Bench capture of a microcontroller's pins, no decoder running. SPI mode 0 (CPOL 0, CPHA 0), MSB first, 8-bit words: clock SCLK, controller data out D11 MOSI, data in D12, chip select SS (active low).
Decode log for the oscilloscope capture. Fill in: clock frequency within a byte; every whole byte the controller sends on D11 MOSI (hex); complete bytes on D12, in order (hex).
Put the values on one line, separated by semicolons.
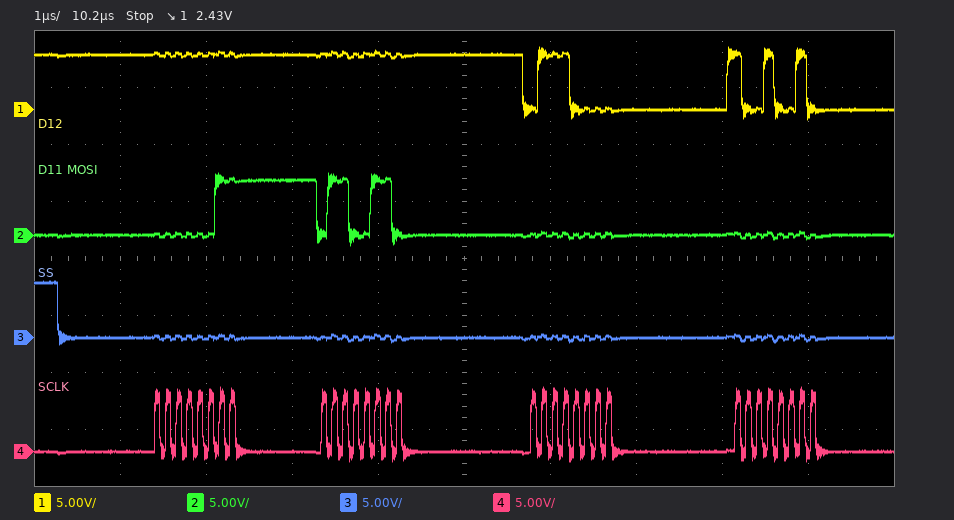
8 MHz; 0x03 0x66 0x00 0x00; 0xFF 0xFF 0x70 0x92
